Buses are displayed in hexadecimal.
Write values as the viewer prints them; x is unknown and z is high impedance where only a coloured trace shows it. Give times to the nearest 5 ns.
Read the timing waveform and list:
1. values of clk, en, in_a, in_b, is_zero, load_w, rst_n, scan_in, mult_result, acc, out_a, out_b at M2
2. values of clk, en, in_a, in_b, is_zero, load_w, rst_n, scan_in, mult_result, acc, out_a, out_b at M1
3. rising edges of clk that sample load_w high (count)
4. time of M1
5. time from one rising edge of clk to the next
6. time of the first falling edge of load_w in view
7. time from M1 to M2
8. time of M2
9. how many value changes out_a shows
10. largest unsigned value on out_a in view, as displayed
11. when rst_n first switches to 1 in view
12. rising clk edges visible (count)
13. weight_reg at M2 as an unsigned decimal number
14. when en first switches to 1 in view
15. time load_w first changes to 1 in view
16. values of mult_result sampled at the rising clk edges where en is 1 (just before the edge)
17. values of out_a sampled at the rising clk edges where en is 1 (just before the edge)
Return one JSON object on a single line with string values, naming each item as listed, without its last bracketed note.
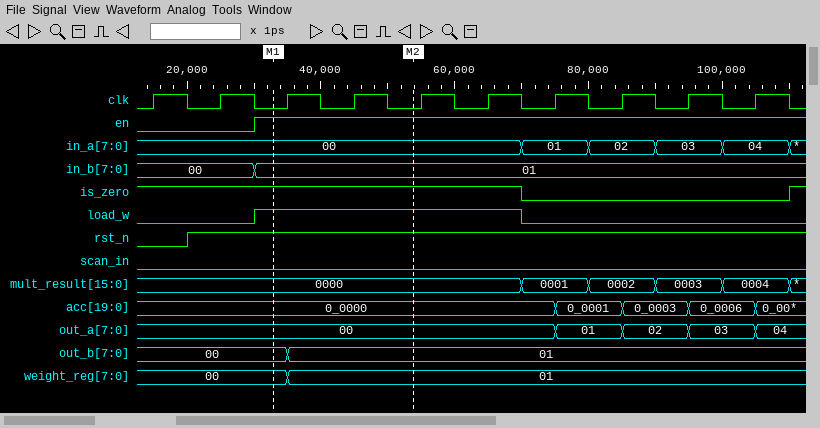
{"values of clk, en, in_a, in_b, is_zero, load_w, rst_n, scan_in, mult_result, acc, out_a, out_b at M2": "clk=0, en=1, in_a=00, in_b=01, is_zero=1, load_w=1, rst_n=1, scan_in=0, mult_result=0000, acc=0_0000, out_a=00, out_b=01", "values of clk, en, in_a, in_b, is_zero, load_w, rst_n, scan_in, mult_result, acc, out_a, out_b at M1": "clk=0, en=1, in_a=00, in_b=01, is_zero=1, load_w=1, rst_n=1, scan_in=0, mult_result=0000, acc=0_0000, out_a=00, out_b=00", "rising edges of clk that sample load_w high": "4", "time of M1": "35 ns", "time from one rising edge of clk to the next": "10 ns", "time of the first falling edge of load_w in view": "70 ns", "time from M1 to M2": "20 ns", "time of M2": "55 ns", "how many value changes out_a shows": "4", "largest unsigned value on out_a in view, as displayed": "04", "when rst_n first switches to 1 in view": "20 ns", "rising clk edges visible": "10", "weight_reg at M2 as an unsigned decimal number": "1", "when en first switches to 1 in view": "30 ns", "time load_w first changes to 1 in view": "30 ns", "values of mult_result sampled at the rising clk edges where en is 1": "0000, 0000, 0000, 0000, 0001, 0002, 0003, 0004", "values of out_a sampled at the rising clk edges where en is 1": "00, 00, 00, 00, 00, 01, 02, 03"}
